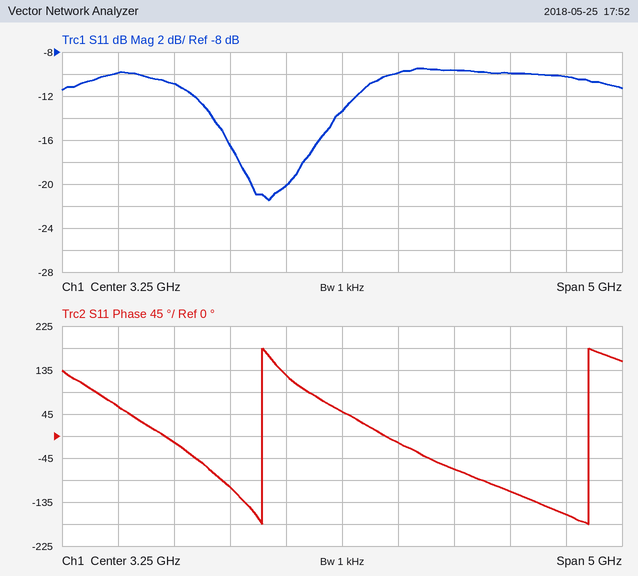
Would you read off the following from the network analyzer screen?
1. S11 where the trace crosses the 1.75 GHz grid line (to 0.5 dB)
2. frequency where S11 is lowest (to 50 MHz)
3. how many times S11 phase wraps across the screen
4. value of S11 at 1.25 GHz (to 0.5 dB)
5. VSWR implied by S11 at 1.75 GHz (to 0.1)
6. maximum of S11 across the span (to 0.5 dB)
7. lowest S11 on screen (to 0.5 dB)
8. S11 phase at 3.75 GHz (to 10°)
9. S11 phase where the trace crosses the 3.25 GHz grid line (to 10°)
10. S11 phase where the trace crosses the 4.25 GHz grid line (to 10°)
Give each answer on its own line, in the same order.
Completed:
-11.0 dB
2.60 GHz
2
-10.0 dB
1.8
-9.5 dB
-21.5 dB
-10°
50°
-70°
